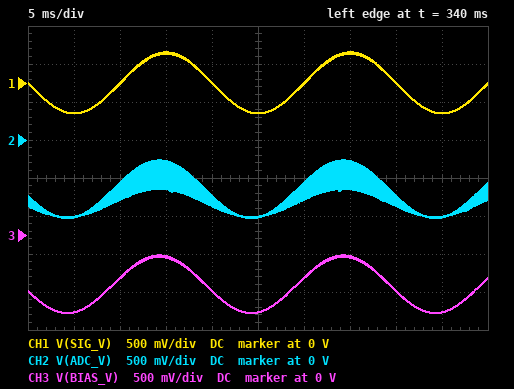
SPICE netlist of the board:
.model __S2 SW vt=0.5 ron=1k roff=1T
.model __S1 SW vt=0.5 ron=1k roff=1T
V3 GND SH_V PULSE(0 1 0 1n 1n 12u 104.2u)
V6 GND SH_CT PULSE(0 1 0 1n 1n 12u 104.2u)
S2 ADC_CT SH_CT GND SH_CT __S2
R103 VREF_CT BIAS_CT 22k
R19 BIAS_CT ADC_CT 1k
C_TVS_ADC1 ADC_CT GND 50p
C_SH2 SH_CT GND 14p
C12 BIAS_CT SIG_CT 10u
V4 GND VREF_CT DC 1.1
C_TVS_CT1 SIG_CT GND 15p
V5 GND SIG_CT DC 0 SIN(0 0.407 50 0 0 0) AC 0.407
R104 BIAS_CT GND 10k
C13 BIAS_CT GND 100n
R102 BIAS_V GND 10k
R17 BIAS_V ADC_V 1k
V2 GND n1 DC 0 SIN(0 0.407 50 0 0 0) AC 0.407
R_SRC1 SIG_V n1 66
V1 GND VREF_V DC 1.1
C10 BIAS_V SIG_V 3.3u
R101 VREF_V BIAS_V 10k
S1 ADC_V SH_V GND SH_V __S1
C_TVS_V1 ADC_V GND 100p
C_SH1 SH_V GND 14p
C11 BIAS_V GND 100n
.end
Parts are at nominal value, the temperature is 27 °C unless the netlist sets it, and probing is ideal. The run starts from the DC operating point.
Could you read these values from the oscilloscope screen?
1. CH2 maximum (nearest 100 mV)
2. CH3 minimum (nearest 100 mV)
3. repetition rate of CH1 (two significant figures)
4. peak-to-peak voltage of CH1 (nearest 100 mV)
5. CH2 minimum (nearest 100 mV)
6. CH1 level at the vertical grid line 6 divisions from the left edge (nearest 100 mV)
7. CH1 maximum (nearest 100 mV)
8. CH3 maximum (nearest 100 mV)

-300 mV
-1.0 V
50 Hz
800 mV
-1.0 V
0 V
400 mV
-300 mV
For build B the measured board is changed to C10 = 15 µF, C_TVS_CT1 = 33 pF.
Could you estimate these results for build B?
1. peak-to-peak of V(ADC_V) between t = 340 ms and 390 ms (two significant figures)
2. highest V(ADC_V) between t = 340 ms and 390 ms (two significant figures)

800 mV
-250 mV
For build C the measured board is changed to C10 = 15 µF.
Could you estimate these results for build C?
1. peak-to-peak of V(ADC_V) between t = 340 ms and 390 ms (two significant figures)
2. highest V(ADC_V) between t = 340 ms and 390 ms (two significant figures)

800 mV
-250 mV
